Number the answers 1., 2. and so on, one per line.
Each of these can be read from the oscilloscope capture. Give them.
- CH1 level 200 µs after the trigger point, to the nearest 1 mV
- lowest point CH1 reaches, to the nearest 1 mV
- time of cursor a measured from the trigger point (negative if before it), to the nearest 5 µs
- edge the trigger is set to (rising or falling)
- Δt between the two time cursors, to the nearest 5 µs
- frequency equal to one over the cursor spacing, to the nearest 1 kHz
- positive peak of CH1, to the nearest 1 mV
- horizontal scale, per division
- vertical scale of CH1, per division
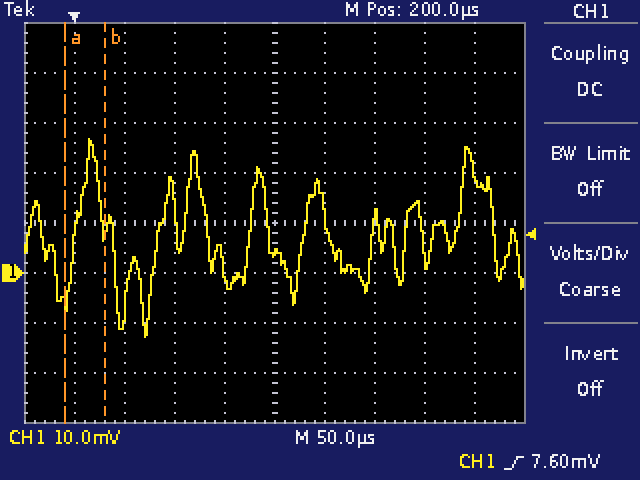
1. 4 mV
2. -13 mV
3. -10 µs
4. rising
5. 40 µs
6. 25 kHz
7. 27 mV
8. 50 µs
9. 10 mV
